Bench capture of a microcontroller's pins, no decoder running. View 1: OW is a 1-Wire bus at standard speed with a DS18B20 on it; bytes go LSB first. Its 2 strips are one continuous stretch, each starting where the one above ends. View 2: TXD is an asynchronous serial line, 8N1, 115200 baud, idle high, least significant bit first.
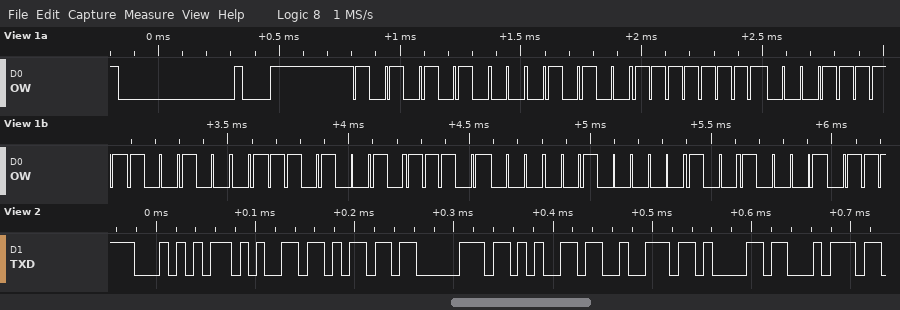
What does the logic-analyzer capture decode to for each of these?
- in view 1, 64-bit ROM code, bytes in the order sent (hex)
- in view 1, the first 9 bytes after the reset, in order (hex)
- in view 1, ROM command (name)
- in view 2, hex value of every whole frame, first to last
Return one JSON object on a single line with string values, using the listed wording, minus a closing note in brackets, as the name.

{"in view 1, 64-bit ROM code, bytes in the order sent": "28 FF F8 89 4B 17 04 89", "in view 1, the first 9 bytes after the reset, in order": "55 28 FF F8 89 4B 17 04 89", "in view 1, ROM command": "Match ROM", "in view 2, hex value of every whole frame, first to last": "54 65 6D 70 65 72 61 74"}
